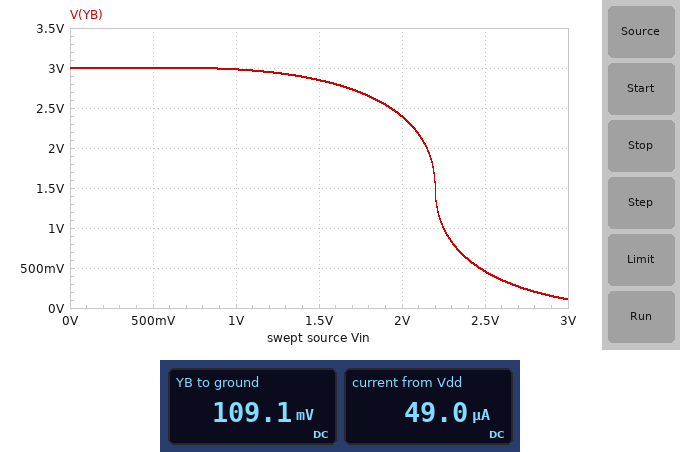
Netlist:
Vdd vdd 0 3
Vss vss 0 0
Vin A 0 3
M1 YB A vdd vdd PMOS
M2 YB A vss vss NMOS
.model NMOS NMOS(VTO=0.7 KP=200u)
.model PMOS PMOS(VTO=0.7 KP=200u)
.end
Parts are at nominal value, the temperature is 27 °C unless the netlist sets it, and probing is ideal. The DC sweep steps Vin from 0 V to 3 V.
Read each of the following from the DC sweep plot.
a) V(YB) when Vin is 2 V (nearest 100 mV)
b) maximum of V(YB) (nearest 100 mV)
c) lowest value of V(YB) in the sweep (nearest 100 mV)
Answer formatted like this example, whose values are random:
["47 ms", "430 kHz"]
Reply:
["2.4 V", "3.0 V", "100 mV"]
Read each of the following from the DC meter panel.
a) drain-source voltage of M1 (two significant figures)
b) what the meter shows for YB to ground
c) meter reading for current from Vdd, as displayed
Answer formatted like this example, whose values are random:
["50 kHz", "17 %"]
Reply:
["-2.9 V", "109.1 mV", "49.0 µA"]
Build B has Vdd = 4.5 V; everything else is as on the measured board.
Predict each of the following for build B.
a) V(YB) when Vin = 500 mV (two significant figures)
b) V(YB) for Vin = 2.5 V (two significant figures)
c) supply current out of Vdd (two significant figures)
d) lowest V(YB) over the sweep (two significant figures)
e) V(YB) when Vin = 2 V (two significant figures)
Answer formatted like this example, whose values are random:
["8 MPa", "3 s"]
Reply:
["4.5 V", "3.8 V", "480 µA", "1.6 V", "4.2 V"]
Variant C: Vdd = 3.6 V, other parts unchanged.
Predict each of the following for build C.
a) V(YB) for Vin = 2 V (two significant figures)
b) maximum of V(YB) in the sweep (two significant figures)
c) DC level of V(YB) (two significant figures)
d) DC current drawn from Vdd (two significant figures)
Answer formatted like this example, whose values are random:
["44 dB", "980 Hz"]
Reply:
["3.2 V", "3.6 V", "400 mV", "170 µA"]
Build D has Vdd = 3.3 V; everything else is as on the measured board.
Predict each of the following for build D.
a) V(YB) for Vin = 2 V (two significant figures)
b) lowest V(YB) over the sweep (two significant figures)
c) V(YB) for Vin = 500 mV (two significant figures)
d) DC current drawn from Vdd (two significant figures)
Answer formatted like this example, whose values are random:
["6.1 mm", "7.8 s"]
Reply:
["2.8 V", "230 mV", "3.3 V", "100 µA"]
